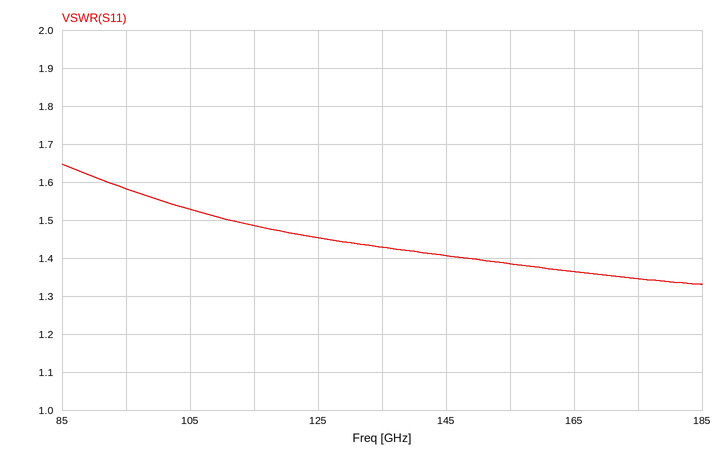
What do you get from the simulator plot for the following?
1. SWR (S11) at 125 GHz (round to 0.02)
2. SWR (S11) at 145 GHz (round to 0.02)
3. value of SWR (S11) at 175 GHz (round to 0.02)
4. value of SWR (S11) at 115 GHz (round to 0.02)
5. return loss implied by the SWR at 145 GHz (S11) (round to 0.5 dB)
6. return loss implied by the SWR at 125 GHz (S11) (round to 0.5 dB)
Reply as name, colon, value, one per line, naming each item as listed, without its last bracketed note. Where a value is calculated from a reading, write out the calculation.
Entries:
SWR (S11) at 125 GHz: 1.46
SWR (S11) at 145 GHz: 1.40
value of SWR (S11) at 175 GHz: 1.34
value of SWR (S11) at 115 GHz: 1.48
return loss implied by the SWR at 145 GHz (S11): −20 log10((1.4 − 1)/(1.4 + 1)) ≈ 15.6 dB, so 15.5 dB to the nearest 0.5 dB
return loss implied by the SWR at 125 GHz (S11): −20 log10((1.46 − 1)/(1.46 + 1)) ≈ 14.6 dB, so 14.5 dB to the nearest 0.5 dB
